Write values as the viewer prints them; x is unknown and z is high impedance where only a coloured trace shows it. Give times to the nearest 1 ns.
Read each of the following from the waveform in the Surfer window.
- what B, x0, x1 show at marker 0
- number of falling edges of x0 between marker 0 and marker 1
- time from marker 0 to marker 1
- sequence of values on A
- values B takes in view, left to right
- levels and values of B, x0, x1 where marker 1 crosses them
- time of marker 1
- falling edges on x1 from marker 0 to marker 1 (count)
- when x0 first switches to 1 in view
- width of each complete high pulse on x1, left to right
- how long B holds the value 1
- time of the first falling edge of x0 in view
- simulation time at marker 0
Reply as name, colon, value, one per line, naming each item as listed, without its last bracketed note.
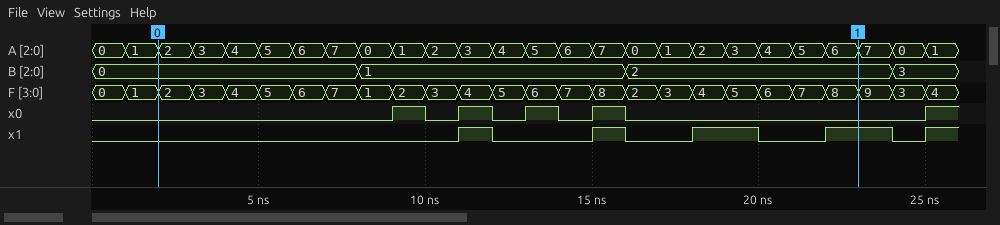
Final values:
what B, x0, x1 show at marker 0: B=0, x0=0, x1=0
number of falling edges of x0 between marker 0 and marker 1: 4
time from marker 0 to marker 1: 21 ns
sequence of values on A: 0, 1, 2, 3, 4, 5, 6, 7, 0, 1, 2, 3, 4, 5, 6, 7, 0, 1, 2, 3, 4, 5, 6, 7, 0, 1
values B takes in view, left to right: 0, 1, 2, 3
levels and values of B, x0, x1 where marker 1 crosses them: B=2, x0=0, x1=1
time of marker 1: 23 ns
falling edges on x1 from marker 0 to marker 1: 3
when x0 first switches to 1 in view: 9 ns
width of each complete high pulse on x1, left to right: 1 ns, 1 ns, 2 ns, 2 ns
how long B holds the value 1: 8 ns
time of the first falling edge of x0 in view: 10 ns
simulation time at marker 0: 2 ns
